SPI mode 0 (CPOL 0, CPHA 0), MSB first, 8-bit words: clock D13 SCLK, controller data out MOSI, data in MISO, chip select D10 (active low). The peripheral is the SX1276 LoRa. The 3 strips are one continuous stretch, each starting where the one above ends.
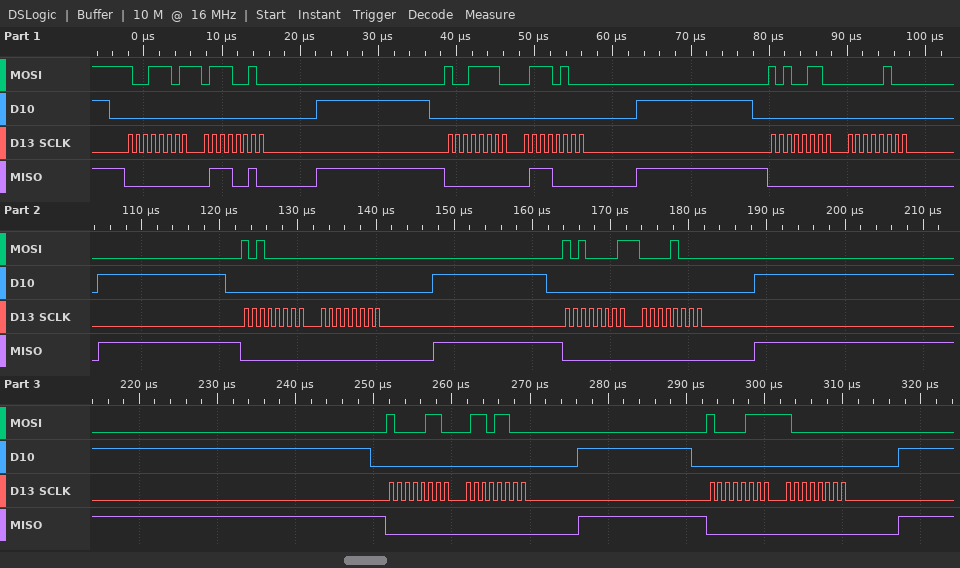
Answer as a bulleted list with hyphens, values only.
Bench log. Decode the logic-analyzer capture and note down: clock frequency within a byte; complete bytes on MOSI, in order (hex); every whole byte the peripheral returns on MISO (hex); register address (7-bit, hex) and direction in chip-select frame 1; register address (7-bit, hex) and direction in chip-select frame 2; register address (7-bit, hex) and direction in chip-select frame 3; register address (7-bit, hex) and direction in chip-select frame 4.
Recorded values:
- 1 MHz
- 9D 72 9E 74 A6 04 A0 00 A1 08 86 6C 87 80
- 00 72 00 70 00 00 00 00 00 00 00 00 00 00
- 0x1D write
- 0x1E write
- 0x26 write
- 0x20 write
